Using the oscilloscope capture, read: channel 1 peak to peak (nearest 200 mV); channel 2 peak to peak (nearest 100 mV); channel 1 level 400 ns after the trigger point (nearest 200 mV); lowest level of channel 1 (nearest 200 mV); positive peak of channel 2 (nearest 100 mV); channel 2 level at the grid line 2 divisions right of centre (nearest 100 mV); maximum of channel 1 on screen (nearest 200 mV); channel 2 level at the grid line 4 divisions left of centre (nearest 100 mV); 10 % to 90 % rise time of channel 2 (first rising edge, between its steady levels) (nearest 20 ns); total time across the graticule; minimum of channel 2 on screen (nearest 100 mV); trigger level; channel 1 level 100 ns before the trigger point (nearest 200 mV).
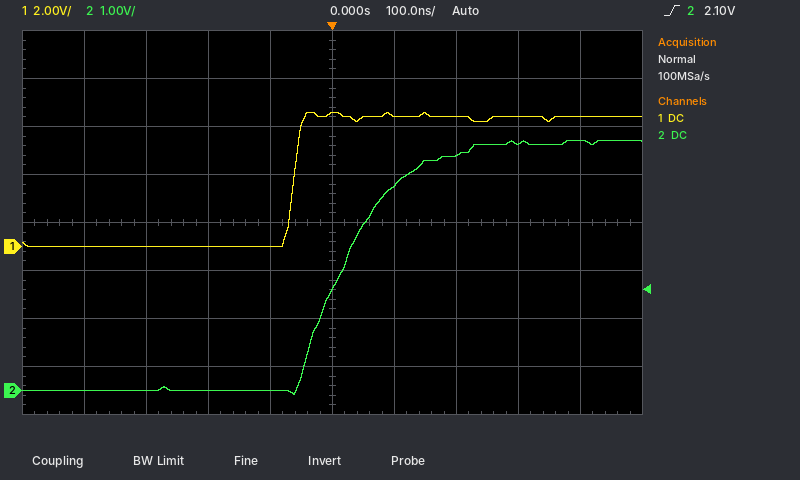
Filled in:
5.6 V
5.3 V
5.4 V
0.0 V
5.2 V
4.9 V
5.6 V
0.0 V
180 ns
1 µs
-100 mV
2.10 V
0.0 V
